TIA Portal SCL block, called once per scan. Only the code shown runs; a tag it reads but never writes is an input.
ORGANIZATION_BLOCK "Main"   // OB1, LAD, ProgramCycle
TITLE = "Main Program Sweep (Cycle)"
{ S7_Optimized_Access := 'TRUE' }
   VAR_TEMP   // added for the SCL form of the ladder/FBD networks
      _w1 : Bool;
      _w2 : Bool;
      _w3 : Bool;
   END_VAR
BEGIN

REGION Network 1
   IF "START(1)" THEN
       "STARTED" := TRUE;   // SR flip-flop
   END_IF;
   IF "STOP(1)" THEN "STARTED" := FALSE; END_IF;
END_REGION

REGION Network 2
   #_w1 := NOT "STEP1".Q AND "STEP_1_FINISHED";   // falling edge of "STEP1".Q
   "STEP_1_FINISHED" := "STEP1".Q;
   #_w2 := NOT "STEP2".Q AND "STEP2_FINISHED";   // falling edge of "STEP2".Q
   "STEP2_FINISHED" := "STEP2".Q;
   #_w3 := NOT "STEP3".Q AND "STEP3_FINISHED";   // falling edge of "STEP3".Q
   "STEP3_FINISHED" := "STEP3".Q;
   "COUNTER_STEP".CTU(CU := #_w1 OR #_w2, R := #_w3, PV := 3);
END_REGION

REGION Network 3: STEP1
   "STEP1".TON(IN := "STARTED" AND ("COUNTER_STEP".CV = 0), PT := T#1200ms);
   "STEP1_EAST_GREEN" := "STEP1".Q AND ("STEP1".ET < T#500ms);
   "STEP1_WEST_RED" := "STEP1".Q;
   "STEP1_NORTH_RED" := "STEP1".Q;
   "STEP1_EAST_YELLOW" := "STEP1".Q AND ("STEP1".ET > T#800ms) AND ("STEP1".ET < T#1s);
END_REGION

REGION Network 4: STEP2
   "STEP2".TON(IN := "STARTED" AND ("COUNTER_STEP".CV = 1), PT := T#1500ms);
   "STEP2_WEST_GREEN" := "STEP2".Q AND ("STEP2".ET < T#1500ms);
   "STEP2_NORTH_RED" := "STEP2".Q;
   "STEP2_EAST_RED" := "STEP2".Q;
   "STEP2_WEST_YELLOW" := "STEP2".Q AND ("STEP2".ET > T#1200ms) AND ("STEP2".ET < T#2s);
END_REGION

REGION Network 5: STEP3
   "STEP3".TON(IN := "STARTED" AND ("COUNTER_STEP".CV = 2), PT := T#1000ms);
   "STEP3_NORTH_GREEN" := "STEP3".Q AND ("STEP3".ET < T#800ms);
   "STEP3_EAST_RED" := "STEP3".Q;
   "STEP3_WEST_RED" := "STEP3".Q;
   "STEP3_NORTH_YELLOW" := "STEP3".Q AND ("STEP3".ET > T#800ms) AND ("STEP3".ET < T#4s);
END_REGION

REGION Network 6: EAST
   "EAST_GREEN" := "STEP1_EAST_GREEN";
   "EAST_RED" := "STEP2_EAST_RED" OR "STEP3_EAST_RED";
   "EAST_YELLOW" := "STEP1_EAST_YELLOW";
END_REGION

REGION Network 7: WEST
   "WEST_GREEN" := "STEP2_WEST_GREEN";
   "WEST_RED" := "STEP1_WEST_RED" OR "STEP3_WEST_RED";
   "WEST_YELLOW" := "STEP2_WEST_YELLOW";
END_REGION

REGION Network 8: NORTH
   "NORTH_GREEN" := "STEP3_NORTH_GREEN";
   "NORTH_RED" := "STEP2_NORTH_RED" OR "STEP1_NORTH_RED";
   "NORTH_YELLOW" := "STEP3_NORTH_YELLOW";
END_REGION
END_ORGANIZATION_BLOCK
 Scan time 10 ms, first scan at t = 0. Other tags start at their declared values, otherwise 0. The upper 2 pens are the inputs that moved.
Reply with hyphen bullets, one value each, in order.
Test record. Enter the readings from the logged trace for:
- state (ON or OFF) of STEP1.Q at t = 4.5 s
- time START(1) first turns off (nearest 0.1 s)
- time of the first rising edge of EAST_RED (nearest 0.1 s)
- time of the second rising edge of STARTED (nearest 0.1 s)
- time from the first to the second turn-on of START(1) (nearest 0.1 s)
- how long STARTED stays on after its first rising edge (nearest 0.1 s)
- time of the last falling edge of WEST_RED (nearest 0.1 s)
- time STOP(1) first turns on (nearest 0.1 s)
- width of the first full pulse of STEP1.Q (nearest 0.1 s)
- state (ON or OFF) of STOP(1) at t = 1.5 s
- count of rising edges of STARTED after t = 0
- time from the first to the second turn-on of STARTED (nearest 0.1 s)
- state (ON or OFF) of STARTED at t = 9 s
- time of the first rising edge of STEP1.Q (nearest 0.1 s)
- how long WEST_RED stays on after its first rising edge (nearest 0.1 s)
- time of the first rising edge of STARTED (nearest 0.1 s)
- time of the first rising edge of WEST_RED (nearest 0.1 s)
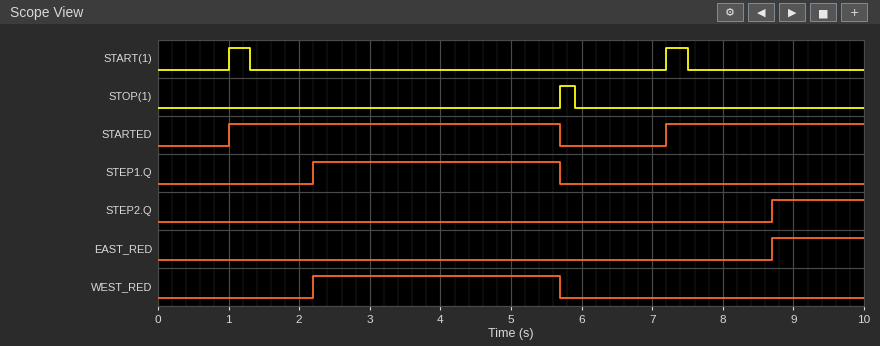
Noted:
- ON
- 1.3 s
- 8.7 s
- 7.2 s
- 6.2 s
- 4.7 s
- 5.7 s
- 5.7 s
- 3.5 s
- OFF
- 2
- 6.2 s
- ON
- 2.2 s
- 3.5 s
- 1.0 s
- 2.2 s
